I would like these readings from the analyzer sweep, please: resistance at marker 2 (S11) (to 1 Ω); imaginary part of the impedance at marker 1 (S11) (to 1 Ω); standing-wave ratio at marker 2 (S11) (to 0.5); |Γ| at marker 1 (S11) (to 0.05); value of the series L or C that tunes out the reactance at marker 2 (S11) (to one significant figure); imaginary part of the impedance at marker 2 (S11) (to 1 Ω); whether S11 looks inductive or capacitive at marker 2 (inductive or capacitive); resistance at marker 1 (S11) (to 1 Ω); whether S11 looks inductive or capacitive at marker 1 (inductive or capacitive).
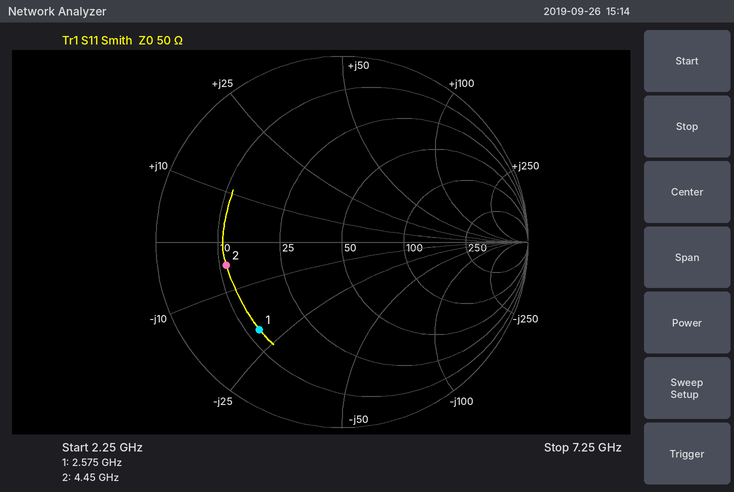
11 Ω
-20 Ω
4.5
0.65
200 pH
-5 Ω
capacitive
13 Ω
capacitive
